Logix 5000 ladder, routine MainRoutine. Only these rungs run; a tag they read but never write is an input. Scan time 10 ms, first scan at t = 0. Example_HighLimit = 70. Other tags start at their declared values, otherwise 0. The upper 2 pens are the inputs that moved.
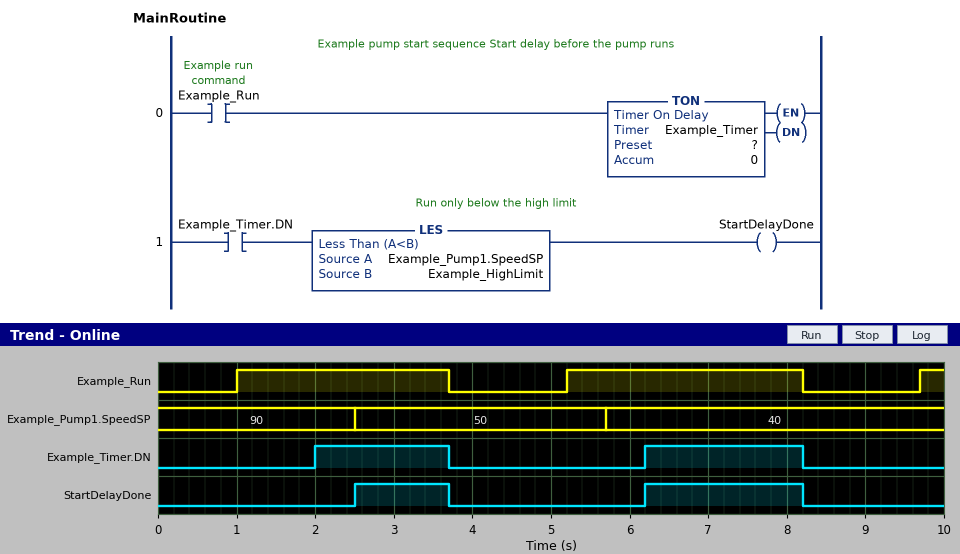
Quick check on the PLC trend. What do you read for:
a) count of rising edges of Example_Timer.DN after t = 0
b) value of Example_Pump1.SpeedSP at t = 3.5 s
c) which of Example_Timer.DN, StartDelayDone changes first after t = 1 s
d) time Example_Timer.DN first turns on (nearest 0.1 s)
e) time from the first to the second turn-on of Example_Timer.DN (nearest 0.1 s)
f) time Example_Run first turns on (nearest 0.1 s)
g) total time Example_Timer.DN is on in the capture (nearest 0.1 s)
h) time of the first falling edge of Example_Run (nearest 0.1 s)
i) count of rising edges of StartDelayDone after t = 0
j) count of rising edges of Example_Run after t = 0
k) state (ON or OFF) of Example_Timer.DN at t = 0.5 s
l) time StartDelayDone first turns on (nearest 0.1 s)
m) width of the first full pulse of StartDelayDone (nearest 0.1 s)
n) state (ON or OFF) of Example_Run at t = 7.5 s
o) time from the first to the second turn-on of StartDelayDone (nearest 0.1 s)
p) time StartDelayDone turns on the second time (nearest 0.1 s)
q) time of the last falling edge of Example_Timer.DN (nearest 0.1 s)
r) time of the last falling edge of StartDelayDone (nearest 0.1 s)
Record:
2
50
Example_Timer.DN
2.0 s
4.2 s
1.0 s
3.7 s
3.7 s
2
3
OFF
2.5 s
1.2 s
ON
3.7 s
6.2 s
8.2 s
8.2 s
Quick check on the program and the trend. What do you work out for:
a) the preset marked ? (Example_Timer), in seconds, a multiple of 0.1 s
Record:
1.0 s
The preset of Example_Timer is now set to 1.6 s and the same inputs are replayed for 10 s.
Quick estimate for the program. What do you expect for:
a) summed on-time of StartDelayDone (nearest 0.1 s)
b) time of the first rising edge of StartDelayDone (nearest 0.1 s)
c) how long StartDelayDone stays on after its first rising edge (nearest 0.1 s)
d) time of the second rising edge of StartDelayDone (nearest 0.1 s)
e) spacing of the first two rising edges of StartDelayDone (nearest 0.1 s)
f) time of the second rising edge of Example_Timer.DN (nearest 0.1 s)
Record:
2.5 s
2.6 s
1.1 s
6.8 s
4.2 s
6.8 s
